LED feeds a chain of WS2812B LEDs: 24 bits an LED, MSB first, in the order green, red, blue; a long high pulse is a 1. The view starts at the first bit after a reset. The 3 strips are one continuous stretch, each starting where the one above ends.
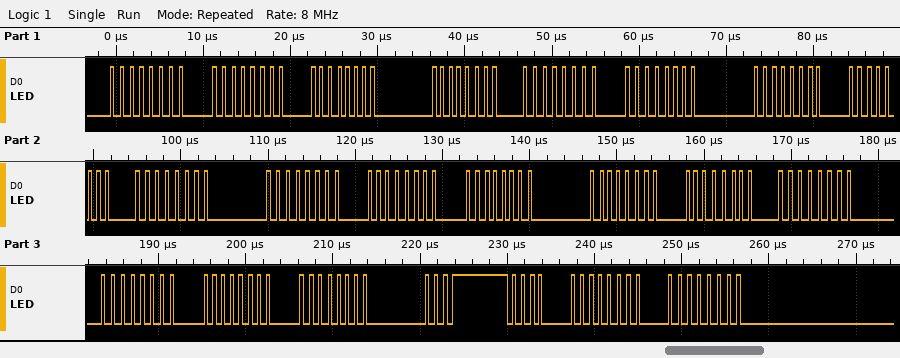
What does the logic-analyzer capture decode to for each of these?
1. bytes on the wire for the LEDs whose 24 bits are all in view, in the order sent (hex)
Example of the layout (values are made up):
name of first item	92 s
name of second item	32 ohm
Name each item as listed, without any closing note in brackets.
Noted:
bytes on the wire for the LEDs whose 24 bits are all in view, in the order sent	00 00 00 00 00 00 00 00 00 00 00 00 00 00 00 00 00 00 10 00 00
